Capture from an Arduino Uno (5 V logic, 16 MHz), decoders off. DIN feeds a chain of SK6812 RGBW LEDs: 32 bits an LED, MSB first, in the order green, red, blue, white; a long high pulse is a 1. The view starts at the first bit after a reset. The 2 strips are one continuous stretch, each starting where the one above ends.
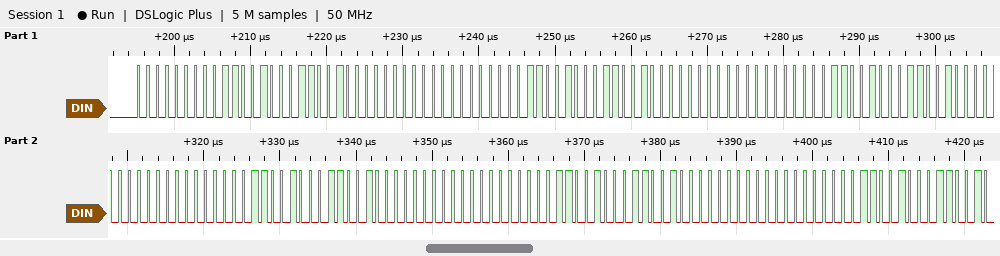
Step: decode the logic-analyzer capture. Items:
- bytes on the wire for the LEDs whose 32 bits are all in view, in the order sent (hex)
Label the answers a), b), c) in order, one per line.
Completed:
a) 00 64 64 00 00 64 64 00 00 64 64 00 00 64 64 00 00 64 64 00
